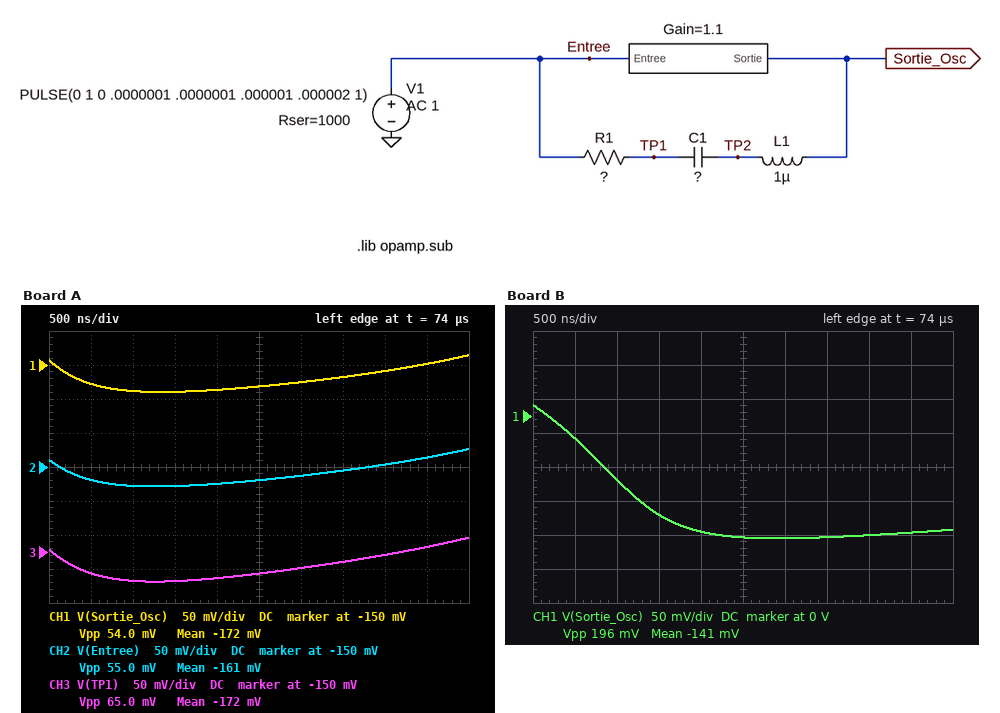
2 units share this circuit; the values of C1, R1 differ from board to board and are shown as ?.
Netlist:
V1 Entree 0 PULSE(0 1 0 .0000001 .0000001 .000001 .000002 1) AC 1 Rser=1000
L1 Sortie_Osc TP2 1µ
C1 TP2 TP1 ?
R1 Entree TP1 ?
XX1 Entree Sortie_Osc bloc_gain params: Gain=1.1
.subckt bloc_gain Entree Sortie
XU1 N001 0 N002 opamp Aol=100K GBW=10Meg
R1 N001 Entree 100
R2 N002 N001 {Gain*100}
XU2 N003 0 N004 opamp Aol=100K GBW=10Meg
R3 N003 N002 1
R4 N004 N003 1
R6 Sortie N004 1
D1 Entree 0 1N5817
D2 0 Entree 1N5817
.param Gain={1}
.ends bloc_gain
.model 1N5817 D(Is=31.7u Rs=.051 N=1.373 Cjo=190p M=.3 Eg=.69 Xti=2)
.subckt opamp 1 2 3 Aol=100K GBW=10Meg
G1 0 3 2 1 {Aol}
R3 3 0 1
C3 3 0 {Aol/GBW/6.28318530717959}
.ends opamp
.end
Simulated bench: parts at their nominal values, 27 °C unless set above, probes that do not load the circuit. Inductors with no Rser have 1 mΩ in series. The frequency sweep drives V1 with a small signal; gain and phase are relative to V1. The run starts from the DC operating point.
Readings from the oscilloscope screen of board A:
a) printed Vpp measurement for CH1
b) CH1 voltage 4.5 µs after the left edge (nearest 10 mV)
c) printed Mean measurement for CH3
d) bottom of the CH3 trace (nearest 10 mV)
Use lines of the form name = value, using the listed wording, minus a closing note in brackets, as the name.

printed Vpp measurement for CH1 = 54.0 mV
CH1 voltage 4.5 µs after the left edge = -150 mV
printed Mean measurement for CH3 = -172 mV
bottom of the CH3 trace = -190 mV
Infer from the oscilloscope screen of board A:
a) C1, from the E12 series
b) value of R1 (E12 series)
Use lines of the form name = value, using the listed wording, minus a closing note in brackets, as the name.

C1, from the E12 series = 1.5 µF
value of R1 = 2.2 Ω
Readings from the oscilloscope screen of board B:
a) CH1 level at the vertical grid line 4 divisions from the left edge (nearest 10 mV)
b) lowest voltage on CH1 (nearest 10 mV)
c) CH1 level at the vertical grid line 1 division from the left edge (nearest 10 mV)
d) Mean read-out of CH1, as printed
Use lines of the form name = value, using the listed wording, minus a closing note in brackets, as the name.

CH1 level at the vertical grid line 4 divisions from the left edge = -170 mV
lowest voltage on CH1 = -180 mV
CH1 level at the vertical grid line 1 division from the left edge = -30 mV
Mean read-out of CH1, as printed = -141 mV
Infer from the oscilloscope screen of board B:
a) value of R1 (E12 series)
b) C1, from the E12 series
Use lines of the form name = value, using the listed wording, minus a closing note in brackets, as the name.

value of R1 = 2.7 Ω
C1, from the E12 series = 2.2 µF
